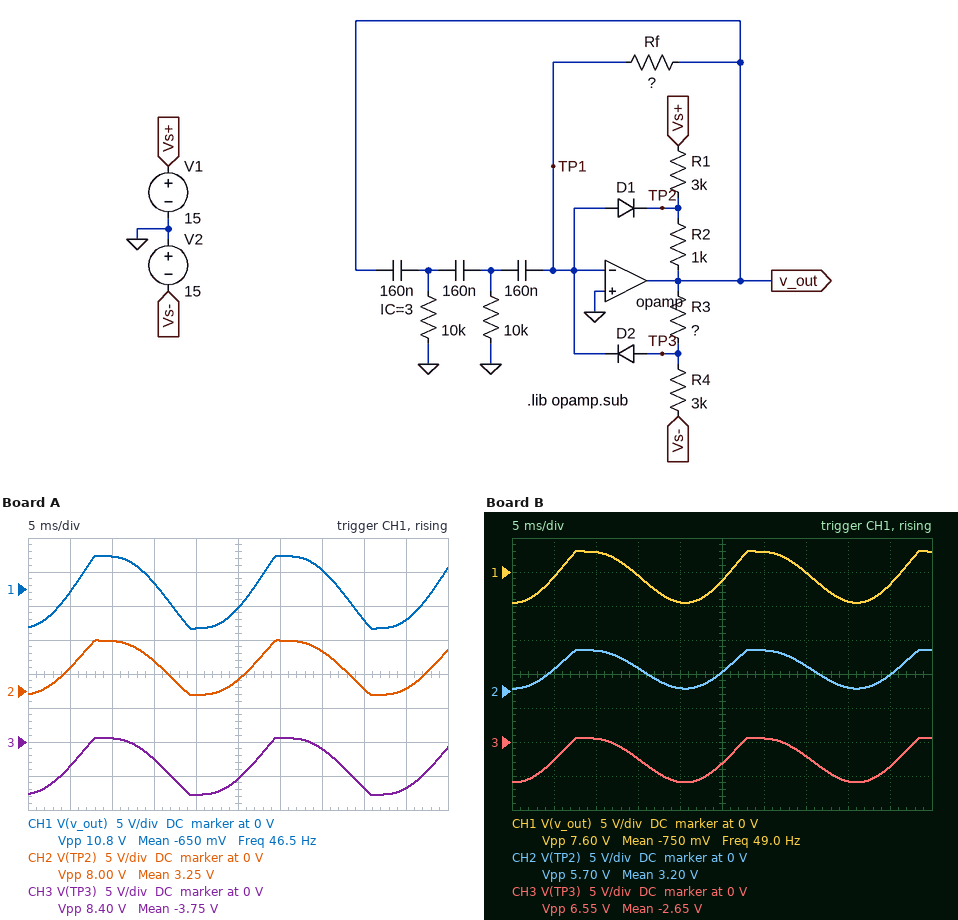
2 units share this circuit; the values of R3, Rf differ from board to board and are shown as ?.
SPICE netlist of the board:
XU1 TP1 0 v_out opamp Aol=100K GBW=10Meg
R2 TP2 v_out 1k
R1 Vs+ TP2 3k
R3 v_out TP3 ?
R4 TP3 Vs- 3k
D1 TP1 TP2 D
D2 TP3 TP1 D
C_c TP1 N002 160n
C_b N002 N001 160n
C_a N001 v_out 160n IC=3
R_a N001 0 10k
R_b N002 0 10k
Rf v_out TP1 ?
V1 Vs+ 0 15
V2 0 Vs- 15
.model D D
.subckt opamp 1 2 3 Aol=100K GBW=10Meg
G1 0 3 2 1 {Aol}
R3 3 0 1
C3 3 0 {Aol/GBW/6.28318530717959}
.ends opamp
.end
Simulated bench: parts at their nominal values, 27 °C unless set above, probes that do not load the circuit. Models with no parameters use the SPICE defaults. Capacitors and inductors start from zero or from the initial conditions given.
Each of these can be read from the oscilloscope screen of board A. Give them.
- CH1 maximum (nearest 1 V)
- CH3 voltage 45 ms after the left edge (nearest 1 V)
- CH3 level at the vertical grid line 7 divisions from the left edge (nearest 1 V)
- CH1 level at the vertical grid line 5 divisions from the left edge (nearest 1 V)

5 V
-7 V
-1 V
-3 V
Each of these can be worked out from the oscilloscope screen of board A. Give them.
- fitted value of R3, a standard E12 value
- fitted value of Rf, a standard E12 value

820 Ω
330 kΩ
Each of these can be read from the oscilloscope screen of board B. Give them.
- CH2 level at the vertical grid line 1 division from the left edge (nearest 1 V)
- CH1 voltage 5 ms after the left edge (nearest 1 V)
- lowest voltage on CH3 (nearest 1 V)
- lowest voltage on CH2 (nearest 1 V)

3 V
-1 V
-6 V
0 V
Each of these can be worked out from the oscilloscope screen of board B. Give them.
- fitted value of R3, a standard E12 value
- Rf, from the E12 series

470 Ω
220 kΩ
